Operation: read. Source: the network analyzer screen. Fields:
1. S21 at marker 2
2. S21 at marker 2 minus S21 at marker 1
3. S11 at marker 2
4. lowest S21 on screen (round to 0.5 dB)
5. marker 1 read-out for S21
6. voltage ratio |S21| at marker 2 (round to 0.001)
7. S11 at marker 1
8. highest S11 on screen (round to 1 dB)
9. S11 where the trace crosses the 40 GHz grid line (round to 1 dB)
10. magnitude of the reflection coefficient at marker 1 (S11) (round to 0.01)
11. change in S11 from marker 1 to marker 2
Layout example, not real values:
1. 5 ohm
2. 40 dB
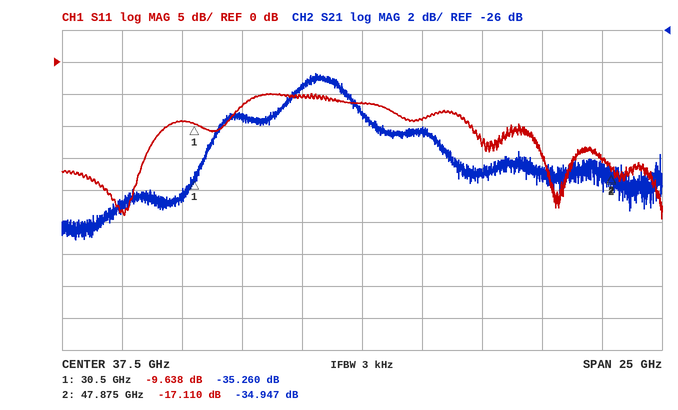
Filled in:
1. -34.947 dB
2. 0.313 dB
3. -17.110 dB
4. -39.0 dB
5. -35.260 dB
6. 0.018
7. -9.638 dB
8. -5 dB
9. -9 dB
10. 0.33
11. -7.472 dB
